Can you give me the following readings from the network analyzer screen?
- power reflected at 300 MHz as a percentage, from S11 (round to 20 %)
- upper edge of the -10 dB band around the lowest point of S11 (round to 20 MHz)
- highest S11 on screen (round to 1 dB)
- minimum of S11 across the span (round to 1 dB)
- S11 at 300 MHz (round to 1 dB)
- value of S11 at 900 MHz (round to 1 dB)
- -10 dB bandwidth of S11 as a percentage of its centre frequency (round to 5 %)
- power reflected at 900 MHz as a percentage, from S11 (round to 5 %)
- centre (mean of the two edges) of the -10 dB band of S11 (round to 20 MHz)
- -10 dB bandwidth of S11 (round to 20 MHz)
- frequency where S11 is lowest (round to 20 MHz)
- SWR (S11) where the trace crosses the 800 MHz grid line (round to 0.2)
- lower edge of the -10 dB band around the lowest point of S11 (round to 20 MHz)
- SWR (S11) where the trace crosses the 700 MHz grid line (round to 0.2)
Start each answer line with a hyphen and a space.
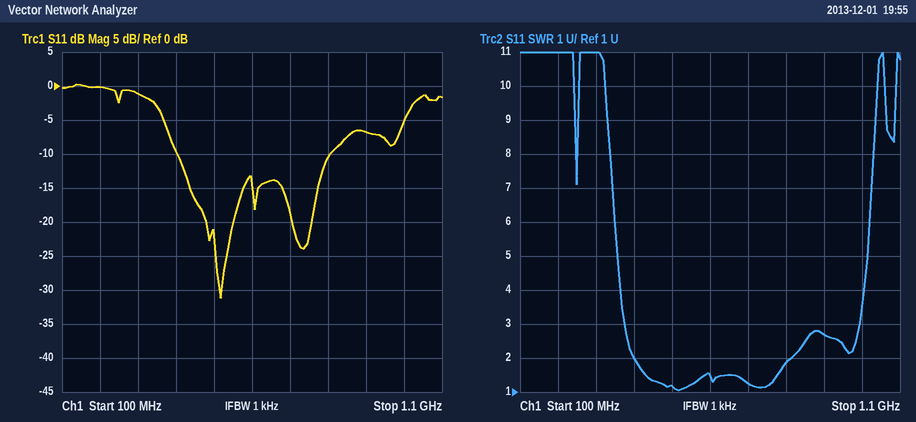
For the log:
- 80 %
- 800 MHz
- 0 dB
- -31 dB
- -1 dB
- -7 dB
- 65 %
- 20 %
- 600 MHz
- 400 MHz
- 520 MHz
- 1.8
- 400 MHz
- 1.2
